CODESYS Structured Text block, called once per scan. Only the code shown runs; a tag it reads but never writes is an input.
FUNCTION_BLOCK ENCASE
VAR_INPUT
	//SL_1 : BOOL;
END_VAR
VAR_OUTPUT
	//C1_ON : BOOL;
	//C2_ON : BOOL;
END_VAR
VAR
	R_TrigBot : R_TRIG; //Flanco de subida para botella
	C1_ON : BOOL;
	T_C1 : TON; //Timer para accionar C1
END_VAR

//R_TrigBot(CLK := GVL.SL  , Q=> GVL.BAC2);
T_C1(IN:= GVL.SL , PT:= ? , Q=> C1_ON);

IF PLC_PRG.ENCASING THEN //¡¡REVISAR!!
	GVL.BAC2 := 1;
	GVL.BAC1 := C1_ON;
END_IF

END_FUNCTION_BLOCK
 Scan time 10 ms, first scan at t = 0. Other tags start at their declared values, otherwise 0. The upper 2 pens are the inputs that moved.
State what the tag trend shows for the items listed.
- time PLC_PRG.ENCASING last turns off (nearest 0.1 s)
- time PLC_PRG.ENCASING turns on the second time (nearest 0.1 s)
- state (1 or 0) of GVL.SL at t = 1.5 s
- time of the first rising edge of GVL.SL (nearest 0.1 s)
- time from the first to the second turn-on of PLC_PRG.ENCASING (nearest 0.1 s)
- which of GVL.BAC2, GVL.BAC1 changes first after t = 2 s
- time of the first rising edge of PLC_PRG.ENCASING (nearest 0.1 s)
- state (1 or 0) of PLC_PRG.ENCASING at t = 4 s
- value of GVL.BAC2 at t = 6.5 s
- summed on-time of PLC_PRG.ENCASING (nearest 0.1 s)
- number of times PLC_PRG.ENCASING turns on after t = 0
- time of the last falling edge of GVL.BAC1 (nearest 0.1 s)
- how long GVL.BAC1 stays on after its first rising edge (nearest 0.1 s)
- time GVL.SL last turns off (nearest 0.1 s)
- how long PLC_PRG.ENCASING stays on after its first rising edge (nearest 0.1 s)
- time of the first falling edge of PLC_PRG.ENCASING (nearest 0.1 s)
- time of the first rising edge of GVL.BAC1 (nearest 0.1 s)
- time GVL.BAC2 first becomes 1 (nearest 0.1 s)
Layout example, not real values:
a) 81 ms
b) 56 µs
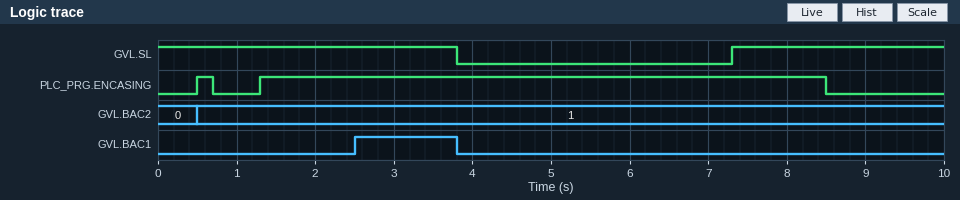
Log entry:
a) 8.5 s
b) 1.3 s
c) 1
d) 7.3 s
e) 0.8 s
f) GVL.BAC1
g) 0.5 s
h) 1
i) 1
j) 7.4 s
k) 2
l) 3.8 s
m) 1.3 s
n) 3.8 s
o) 0.2 s
p) 0.7 s
q) 2.5 s
r) 0.5 s
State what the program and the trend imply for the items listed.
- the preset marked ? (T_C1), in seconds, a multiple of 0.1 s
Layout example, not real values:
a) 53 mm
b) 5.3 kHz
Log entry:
a) 2.5 s
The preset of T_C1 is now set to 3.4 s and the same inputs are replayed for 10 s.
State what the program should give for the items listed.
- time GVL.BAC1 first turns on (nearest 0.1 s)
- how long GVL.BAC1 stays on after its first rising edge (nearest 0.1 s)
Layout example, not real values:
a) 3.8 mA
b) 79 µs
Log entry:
a) 3.4 s
b) 0.4 s
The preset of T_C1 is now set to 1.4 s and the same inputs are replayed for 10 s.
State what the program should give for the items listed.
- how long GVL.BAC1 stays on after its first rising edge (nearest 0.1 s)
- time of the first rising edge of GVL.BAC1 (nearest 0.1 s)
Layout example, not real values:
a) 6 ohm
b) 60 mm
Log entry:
a) 2.4 s
b) 1.4 s
